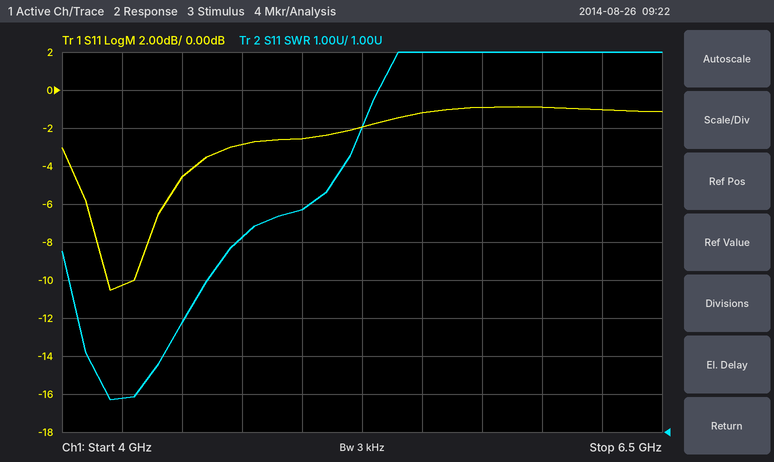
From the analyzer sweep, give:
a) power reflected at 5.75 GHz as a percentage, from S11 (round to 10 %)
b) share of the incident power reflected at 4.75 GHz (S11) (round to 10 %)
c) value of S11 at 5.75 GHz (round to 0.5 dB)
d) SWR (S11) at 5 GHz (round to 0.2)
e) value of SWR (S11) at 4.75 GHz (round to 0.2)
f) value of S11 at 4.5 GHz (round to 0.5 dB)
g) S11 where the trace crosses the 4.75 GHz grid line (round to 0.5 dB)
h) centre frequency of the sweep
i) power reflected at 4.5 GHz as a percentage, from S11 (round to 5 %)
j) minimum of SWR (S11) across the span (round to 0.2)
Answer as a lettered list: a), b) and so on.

a) 80 %
b) 50 %
c) -1.0 dB
d) 6.8
e) 6.2
f) -4.5 dB
g) -3.0 dB
h) 5.25 GHz
i) 35 %
j) 1.8
